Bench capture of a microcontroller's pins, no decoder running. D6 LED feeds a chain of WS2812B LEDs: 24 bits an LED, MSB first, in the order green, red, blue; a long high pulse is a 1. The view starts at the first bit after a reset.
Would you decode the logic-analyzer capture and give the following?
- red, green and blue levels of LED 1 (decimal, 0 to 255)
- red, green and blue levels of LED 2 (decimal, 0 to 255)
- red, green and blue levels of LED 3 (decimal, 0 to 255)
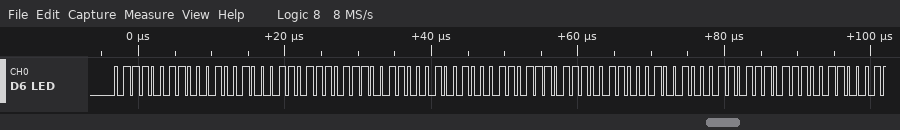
18, 115, 55
18, 115, 55
18, 115, 55
